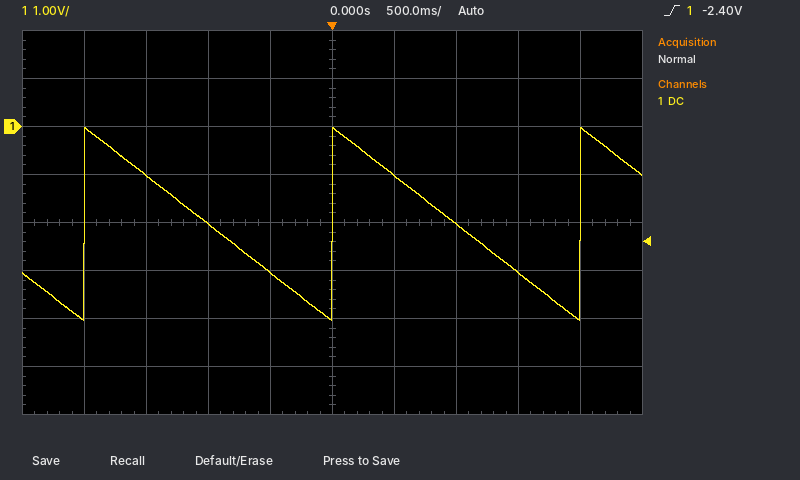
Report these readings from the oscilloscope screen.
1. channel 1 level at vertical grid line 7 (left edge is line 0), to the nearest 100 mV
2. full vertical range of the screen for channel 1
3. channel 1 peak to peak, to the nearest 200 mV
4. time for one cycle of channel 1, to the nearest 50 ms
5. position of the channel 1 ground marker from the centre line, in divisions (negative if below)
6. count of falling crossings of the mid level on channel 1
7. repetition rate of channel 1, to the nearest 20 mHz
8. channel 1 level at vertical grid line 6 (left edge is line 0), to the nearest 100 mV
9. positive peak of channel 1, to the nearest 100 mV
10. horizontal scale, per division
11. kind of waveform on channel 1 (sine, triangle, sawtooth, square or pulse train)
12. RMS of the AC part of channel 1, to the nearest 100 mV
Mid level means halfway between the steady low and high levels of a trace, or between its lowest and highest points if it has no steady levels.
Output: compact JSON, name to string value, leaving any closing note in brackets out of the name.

{"channel 1 level at vertical grid line 7 (left edge is line 0), to the nearest 100 mV": "-2.0 V", "full vertical range of the screen for channel 1": "8 V", "channel 1 peak to peak, to the nearest 200 mV": "4.0 V", "time for one cycle of channel 1, to the nearest 50 ms": "2.00 s", "position of the channel 1 ground marker from the centre line, in divisions": "+2.0 div", "count of falling crossings of the mid level on channel 1": "2", "repetition rate of channel 1, to the nearest 20 mHz": "500 mHz", "channel 1 level at vertical grid line 6 (left edge is line 0), to the nearest 100 mV": "-1.0 V", "positive peak of channel 1, to the nearest 100 mV": "0.0 V", "horizontal scale, per division": "500 ms", "kind of waveform on channel 1": "sawtooth", "RMS of the AC part of channel 1, to the nearest 100 mV": "1.2 V"}
